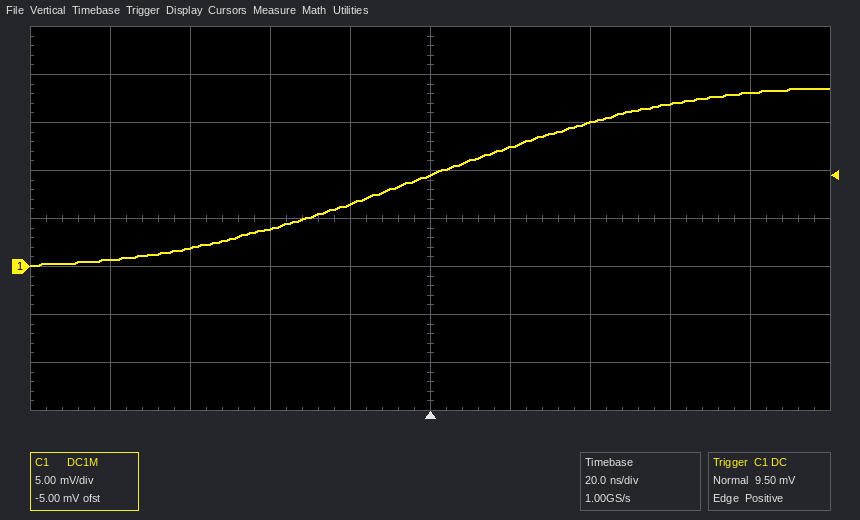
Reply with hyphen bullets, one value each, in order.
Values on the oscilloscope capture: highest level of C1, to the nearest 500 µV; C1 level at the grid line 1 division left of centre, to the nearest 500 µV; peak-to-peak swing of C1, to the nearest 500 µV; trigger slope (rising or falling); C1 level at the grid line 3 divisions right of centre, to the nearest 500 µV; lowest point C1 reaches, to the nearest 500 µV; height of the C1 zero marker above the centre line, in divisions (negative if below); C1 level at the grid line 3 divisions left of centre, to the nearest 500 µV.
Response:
- 18.5 mV
- 6.5 mV
- 18.5 mV
- rising
- 17.0 mV
- 0.0 mV
- -1.0 div
- 2.0 mV
